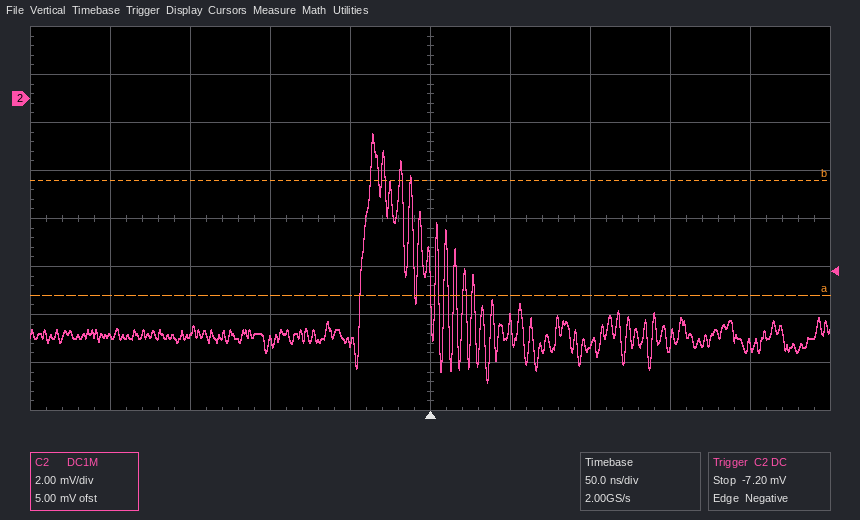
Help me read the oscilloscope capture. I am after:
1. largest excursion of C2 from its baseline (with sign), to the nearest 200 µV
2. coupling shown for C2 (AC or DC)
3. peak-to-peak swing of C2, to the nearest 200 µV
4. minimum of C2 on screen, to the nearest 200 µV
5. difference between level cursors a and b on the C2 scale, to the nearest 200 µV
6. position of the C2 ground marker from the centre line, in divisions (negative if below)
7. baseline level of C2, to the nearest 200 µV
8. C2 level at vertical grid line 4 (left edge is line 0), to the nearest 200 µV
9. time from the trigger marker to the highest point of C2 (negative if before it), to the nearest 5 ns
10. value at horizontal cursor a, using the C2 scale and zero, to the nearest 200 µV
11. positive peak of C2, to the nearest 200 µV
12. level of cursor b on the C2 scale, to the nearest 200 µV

+8.4 mV
DC
10.4 mV
-11.8 mV
4.8 mV
+2.5 div
-9.8 mV
-10.2 mV
-35 ns
-8.2 mV
-1.4 mV
-3.4 mV
